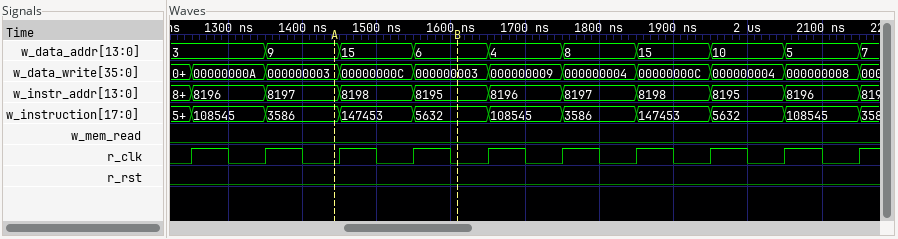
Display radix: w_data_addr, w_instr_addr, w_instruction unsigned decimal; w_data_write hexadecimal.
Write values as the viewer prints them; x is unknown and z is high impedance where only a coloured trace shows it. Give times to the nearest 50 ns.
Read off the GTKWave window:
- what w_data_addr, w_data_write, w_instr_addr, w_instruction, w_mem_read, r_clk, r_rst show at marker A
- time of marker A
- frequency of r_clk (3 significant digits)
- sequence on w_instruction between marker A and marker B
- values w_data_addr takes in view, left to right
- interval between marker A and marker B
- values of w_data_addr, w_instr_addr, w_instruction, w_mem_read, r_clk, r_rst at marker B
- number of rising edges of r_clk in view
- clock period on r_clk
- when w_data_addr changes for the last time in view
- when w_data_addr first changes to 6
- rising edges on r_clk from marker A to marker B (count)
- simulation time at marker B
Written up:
w_data_addr=9, w_data_write=000000003, w_instr_addr=8197, w_instruction=3586, w_mem_read=0, r_clk=0, r_rst=0
1450 ns
10.0 MHz
3586, 147453, 5632
3, 9, 15, 6, 4, 8, 15, 10, 5, 7
150 ns
w_data_addr=6, w_instr_addr=8195, w_instruction=5632, w_mem_read=0, r_clk=0, r_rst=0
10
100 ns
2150 ns
1550 ns
2
1600 ns
